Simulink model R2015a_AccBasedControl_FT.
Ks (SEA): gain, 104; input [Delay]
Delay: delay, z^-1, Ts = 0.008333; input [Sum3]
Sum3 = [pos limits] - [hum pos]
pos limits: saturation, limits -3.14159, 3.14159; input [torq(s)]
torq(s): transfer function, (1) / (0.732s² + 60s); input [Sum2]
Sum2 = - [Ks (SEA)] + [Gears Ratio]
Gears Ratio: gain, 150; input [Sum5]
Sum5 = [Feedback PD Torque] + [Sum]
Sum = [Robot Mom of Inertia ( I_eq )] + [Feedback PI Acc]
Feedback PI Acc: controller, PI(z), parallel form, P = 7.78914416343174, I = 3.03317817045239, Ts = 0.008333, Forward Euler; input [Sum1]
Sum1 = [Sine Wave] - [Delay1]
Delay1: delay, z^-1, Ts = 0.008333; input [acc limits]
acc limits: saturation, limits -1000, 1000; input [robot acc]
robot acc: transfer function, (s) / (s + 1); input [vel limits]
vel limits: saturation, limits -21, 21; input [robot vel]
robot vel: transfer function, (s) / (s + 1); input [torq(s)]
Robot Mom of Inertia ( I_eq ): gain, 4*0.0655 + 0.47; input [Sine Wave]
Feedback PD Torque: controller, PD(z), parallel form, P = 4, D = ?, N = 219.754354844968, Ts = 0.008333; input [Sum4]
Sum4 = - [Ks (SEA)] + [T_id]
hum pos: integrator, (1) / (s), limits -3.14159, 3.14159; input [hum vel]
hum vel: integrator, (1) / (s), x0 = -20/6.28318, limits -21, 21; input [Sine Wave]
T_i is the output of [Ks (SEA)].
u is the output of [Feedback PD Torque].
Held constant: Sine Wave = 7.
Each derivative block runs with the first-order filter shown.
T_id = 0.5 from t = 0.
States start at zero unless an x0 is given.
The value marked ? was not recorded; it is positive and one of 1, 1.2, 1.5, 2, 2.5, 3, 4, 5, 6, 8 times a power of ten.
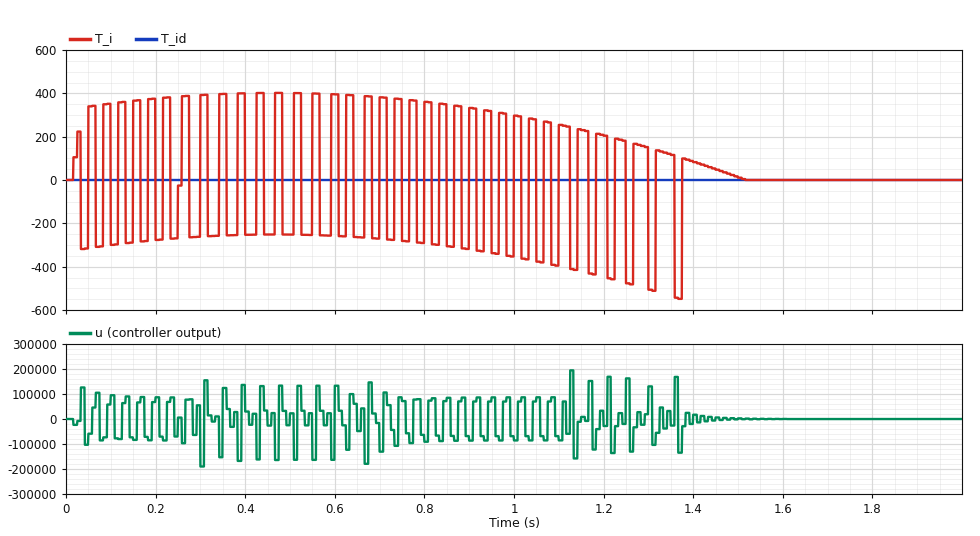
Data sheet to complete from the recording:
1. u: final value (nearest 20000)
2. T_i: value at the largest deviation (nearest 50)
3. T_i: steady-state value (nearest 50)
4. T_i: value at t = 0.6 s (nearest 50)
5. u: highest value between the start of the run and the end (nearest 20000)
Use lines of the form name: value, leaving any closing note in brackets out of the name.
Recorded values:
u: final value: 0
T_i: value at the largest deviation: -550
T_i: steady-state value: 0
T_i: value at t = 0.6 s: 400
u: highest value between the start of the run and the end: 200000
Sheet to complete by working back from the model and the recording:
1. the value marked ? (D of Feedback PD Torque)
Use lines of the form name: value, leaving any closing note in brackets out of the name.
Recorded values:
the value marked ?: 1
